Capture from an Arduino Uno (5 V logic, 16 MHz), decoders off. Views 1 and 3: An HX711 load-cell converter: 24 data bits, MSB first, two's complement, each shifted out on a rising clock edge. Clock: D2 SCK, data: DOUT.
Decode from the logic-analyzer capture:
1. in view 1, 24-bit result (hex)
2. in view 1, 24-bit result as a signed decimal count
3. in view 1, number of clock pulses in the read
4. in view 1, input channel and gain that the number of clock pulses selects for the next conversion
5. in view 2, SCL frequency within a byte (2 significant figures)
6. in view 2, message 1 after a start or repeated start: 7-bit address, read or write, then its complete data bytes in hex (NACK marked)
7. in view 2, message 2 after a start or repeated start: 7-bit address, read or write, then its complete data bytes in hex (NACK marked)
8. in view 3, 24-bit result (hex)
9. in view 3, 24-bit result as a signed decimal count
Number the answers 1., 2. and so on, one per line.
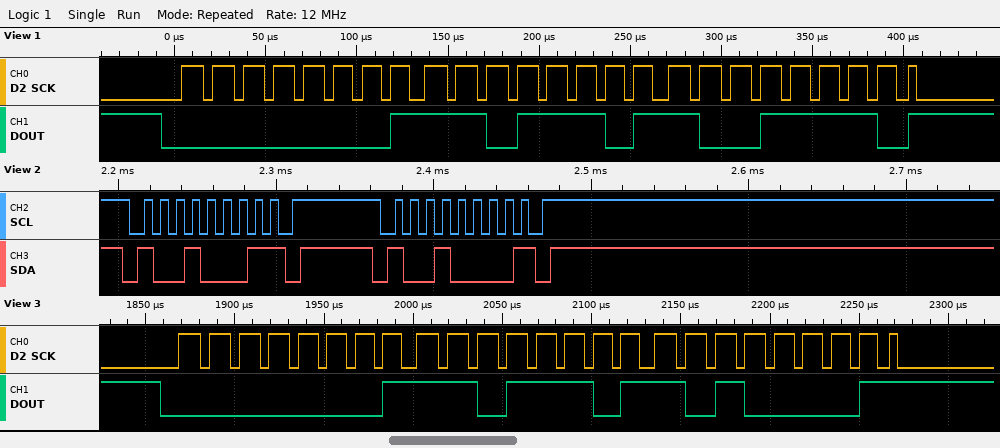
1. 0x01DD9E
2. 122270
3. 25
4. channel A, gain 128
5. 100 kHz
6. 0x48 read NACK
7. 0x48 write NACK
8. 0x01DDA1
9. 122273
